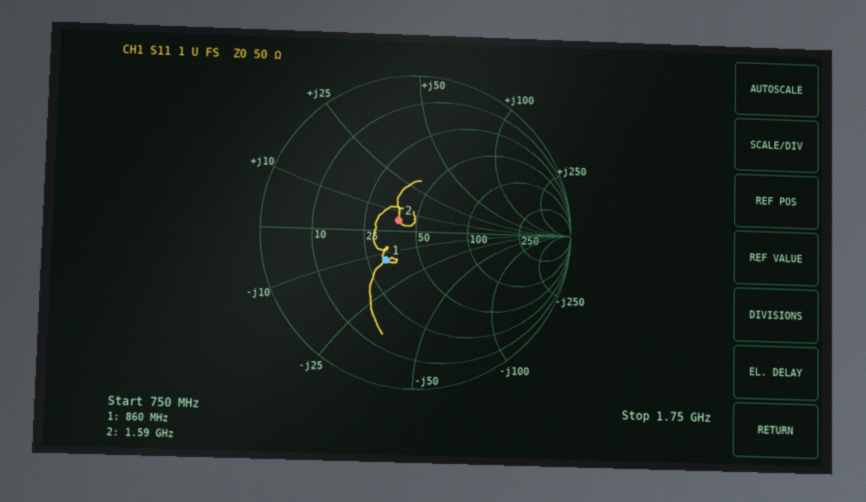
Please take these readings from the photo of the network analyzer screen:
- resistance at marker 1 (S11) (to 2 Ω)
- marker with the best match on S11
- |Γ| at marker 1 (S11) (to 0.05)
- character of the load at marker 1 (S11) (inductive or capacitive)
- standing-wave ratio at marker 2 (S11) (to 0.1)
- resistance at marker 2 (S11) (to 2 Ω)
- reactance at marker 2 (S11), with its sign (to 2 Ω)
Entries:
32 Ω
marker 2
0.25
capacitive
1.3
40 Ω
+6 Ω
